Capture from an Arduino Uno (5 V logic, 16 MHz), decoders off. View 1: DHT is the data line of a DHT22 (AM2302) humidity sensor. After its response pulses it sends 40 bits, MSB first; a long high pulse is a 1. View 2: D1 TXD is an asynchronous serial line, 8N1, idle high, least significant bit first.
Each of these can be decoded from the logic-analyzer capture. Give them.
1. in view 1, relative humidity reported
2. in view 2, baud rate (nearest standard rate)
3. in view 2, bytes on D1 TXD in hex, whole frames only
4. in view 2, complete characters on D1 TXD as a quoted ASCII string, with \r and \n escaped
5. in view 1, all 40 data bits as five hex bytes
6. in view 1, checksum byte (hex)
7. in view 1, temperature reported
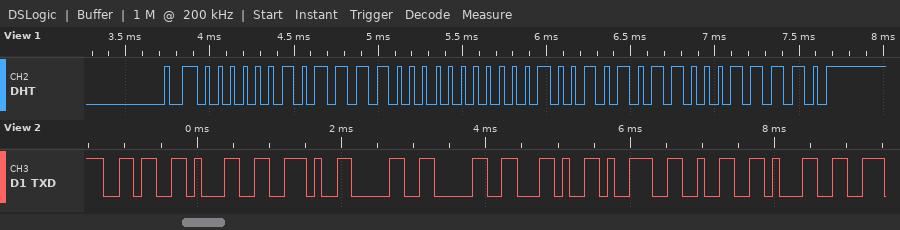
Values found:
75.2 %
9600 baud
0x36 0x31 0x2E 0x30 0x30 0x2C 0x39 0x32 0x31
"61.00,921"
02 F0 01 2B 1E
0x1E
29.9 °C
